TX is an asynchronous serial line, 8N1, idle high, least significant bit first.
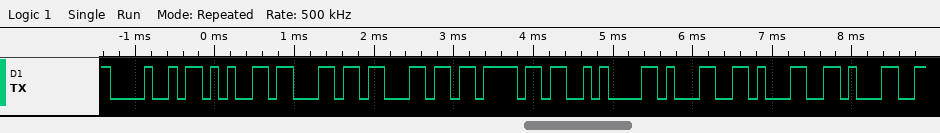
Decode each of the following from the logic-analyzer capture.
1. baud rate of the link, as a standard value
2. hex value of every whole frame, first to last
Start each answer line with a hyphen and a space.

- 9600 baud
- 0x48 0x65 0x6C 0x6C 0x6F 0x0A 0x31 0x31 0x31
